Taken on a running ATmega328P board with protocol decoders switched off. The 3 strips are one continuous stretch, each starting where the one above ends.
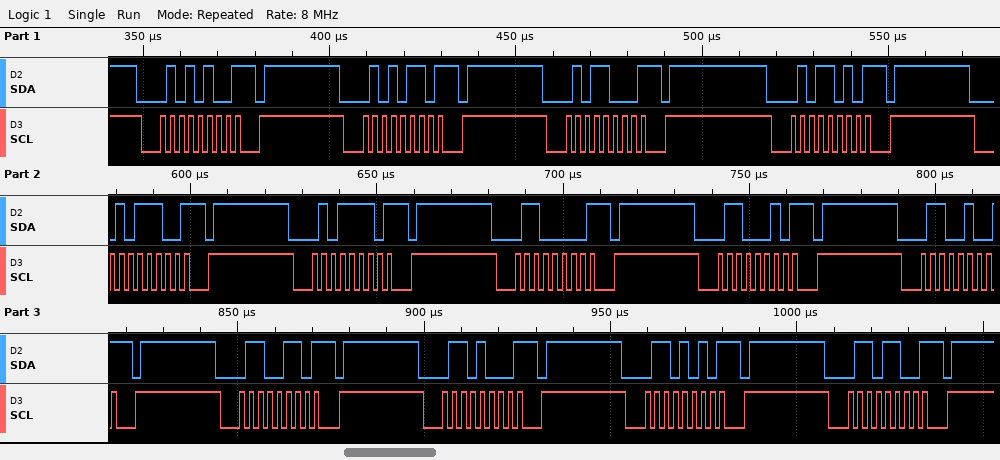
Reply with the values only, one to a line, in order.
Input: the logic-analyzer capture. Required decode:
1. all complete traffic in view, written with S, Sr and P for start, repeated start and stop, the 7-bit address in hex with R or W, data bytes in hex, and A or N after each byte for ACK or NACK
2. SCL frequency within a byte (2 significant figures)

S 2AW N P S 2BW N P S 2CW N P S 2DW N P S 2EW N P S 2FW N P S 30W N P S 31W N P S 32W N P S 33W N P S 34W N P S 35W N P S 36W N P
400 kHz
